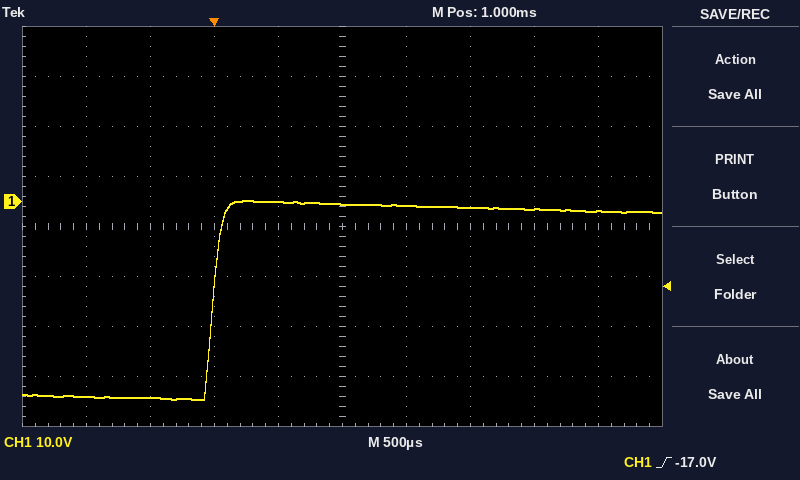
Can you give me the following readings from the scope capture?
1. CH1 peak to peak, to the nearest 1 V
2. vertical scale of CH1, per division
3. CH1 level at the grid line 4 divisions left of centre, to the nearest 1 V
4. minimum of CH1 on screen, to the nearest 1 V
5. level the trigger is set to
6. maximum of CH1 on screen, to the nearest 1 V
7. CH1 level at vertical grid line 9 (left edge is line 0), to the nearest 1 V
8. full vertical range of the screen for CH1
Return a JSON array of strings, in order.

["40 V", "10 V", "-39 V", "-40 V", "-17.0 V", "0 V", "-2 V", "80 V"]
